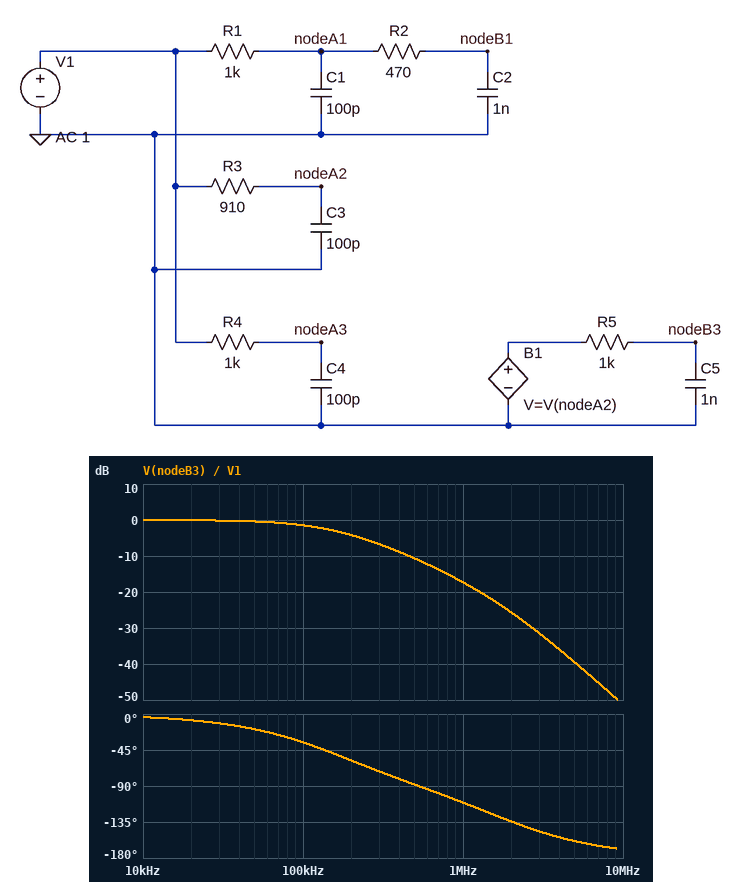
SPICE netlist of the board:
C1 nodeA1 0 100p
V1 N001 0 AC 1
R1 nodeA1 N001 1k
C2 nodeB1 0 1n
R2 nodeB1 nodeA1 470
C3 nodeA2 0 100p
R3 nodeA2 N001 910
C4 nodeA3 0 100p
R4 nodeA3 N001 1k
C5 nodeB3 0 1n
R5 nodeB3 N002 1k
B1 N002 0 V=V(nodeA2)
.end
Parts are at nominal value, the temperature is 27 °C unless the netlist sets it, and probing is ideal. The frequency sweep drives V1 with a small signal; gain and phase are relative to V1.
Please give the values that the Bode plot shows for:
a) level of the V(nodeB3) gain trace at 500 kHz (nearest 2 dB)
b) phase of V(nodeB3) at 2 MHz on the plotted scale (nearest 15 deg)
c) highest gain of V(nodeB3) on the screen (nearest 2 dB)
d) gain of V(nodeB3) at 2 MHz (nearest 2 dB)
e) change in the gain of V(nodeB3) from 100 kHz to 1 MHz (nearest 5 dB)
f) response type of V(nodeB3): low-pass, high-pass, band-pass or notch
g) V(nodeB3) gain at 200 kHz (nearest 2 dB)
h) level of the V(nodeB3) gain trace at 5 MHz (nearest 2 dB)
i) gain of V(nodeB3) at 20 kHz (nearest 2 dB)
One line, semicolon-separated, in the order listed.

-10 dB; -135 deg; 0 dB; -26 dB; -15 dB; low-pass; -4 dB; -40 dB; 0 dB
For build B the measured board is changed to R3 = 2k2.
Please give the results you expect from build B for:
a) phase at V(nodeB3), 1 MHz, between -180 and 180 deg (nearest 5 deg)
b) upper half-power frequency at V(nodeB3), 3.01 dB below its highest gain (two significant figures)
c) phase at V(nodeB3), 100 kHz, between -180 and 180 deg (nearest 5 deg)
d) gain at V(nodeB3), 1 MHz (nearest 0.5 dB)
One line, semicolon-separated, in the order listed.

-135 deg; 150 kHz; -40 deg; -20.5 dB
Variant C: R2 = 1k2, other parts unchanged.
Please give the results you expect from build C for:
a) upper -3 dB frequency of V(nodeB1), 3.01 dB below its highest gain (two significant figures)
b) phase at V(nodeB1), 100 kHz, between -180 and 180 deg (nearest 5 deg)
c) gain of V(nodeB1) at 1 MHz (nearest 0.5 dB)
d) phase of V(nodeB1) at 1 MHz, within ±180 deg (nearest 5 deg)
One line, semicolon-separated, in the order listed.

71 kHz; -55 deg; -23.5 dB; -105 deg
